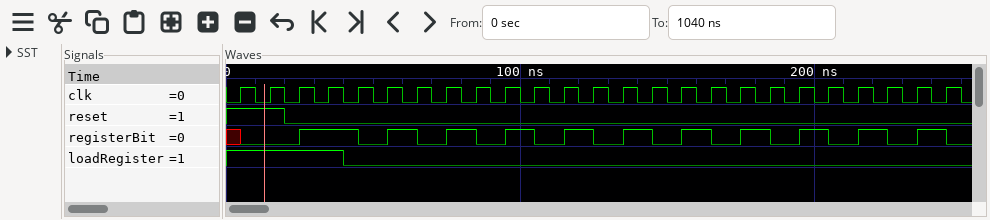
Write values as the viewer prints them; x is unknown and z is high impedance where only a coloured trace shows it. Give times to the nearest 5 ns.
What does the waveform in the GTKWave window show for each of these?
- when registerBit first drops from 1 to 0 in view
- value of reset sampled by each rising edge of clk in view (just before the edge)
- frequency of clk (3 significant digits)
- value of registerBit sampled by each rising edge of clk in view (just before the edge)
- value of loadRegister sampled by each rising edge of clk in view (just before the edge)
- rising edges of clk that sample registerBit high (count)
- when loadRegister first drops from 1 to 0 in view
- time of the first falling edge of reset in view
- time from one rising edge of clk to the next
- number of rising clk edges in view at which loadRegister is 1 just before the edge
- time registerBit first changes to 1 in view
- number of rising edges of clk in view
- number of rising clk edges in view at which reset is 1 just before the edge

45 ns
1 1 0 0 0 0 0 0 0 0 0 0 0 0 0 0 0 0 0 0 0 0 0 0 0
100 MHz
x 0 0 1 1 0 1 0 1 0 1 0 1 0 1 0 1 0 1 0 1 0 1 0 1
1 1 1 1 0 0 0 0 0 0 0 0 0 0 0 0 0 0 0 0 0 0 0 0 0
12
40 ns
20 ns
10 ns
4
25 ns
25
2
